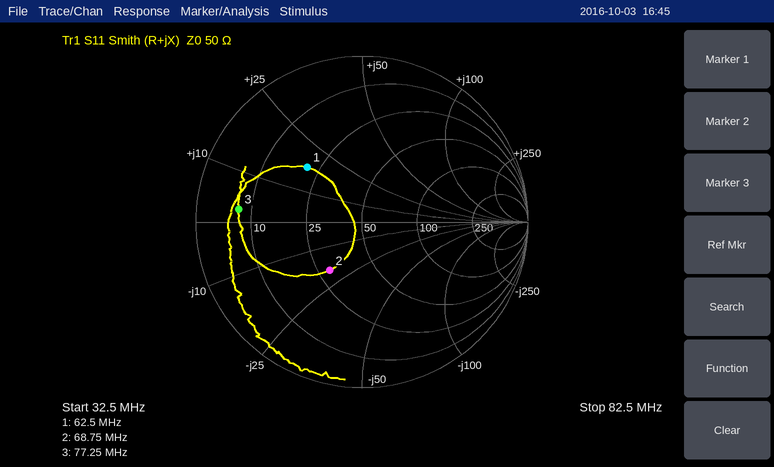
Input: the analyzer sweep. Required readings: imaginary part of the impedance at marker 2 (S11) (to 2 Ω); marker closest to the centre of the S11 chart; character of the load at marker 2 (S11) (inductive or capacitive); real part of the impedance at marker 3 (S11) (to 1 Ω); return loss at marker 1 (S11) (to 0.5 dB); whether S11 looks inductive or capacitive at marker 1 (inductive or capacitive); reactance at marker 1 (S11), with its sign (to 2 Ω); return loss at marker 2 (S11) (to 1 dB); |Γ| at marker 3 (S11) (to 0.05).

-20 Ω
marker 2
capacitive
7 Ω
6.5 dB
inductive
+18 Ω
9 dB
0.75
